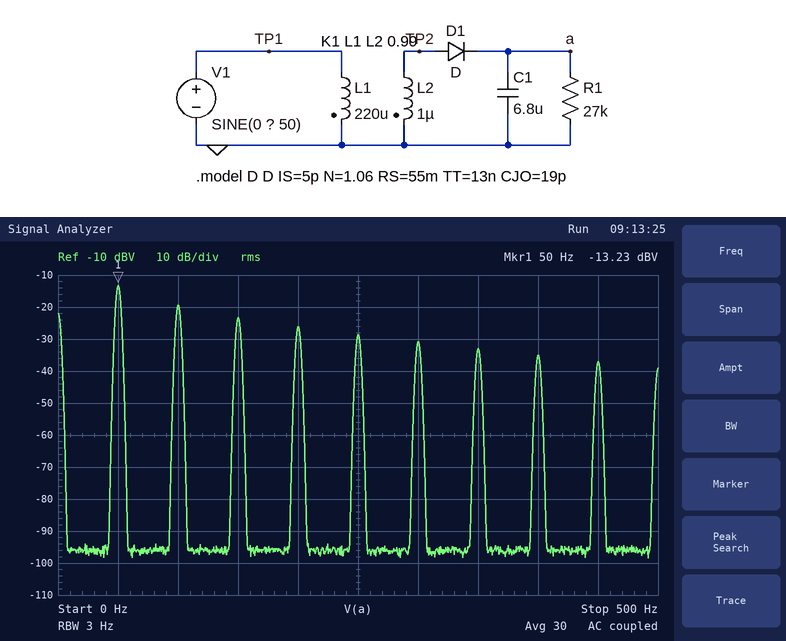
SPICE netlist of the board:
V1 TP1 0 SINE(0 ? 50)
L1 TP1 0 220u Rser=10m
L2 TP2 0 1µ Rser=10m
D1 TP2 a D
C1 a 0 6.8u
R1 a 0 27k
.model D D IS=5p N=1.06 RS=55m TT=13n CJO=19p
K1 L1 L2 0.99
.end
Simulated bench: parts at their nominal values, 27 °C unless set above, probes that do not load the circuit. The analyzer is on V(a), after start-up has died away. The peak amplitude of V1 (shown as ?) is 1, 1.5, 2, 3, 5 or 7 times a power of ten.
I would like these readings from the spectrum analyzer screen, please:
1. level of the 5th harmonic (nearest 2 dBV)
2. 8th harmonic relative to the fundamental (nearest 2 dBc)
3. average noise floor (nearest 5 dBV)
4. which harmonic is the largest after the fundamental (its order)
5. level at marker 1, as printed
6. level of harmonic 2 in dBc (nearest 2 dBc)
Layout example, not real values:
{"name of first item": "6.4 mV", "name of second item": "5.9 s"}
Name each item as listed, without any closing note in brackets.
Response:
{"level of the 5th harmonic": "-28 dBV", "8th harmonic relative to the fundamental": "-22 dBc", "average noise floor": "-95 dBV", "which harmonic is the largest after the fundamental": "2", "level at marker 1, as printed": "-13.23 dBV", "level of harmonic 2 in dBc": "-6 dBc"}
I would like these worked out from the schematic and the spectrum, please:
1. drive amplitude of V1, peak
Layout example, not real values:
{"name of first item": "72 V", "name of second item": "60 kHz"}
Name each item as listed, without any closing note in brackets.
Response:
{"drive amplitude of V1, peak": "150 V"}
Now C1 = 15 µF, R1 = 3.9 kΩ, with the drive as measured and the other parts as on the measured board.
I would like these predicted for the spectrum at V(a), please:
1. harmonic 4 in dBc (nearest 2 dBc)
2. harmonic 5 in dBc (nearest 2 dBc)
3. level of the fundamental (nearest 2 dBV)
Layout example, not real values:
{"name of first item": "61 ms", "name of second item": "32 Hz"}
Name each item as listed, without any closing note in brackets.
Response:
{"harmonic 4 in dBc": "-14 dBc", "harmonic 5 in dBc": "-18 dBc", "level of the fundamental": "-4 dBV"}
